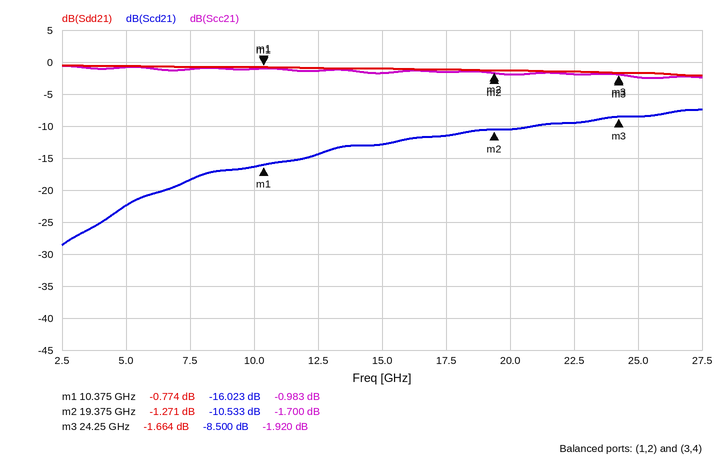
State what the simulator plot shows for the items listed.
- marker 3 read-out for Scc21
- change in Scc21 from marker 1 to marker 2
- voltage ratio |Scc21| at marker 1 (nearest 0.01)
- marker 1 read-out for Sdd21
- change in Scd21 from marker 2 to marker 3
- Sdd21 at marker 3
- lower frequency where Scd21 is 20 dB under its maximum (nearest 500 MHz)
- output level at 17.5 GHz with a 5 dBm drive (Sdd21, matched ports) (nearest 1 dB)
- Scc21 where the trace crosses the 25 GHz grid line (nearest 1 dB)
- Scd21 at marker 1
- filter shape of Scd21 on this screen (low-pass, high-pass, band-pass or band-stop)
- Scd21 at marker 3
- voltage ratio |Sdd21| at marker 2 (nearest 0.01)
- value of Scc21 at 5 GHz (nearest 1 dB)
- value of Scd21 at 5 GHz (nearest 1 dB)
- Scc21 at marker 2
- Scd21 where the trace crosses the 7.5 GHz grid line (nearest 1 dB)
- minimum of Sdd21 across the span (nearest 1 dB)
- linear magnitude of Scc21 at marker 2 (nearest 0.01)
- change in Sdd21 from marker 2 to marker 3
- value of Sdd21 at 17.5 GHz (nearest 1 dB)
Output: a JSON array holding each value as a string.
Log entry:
["-1.920 dB", "-0.717 dB", "0.89", "-0.774 dB", "2.033 dB", "-1.664 dB", "3.0 GHz", "4 dBm", "-2 dB", "-16.023 dB", "high-pass", "-8.500 dB", "0.86", "-1 dB", "-22 dB", "-1.700 dB", "-18 dB", "-2 dB", "0.82", "-0.393 dB", "-1 dB"]
